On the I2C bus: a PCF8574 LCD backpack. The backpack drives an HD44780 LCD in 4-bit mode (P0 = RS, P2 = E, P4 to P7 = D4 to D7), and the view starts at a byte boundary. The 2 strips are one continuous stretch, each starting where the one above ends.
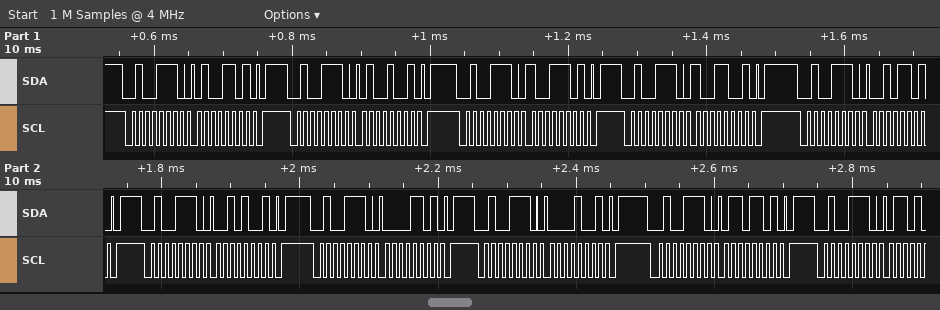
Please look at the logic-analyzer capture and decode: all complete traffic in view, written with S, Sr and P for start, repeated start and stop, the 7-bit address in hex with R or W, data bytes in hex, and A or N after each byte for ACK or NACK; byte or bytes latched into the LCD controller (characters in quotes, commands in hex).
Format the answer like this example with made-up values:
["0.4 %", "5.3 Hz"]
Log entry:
["S 27W A 4D A P S 27W A 49 A P S 27W A 9D A P S 27W A 99 A P S 27W A 2D A P S 27W A 29 A P S 27W A 0D A P S 27W A 09 A P S 27W A 6D A P S 27W A", "'I' ' '"]
